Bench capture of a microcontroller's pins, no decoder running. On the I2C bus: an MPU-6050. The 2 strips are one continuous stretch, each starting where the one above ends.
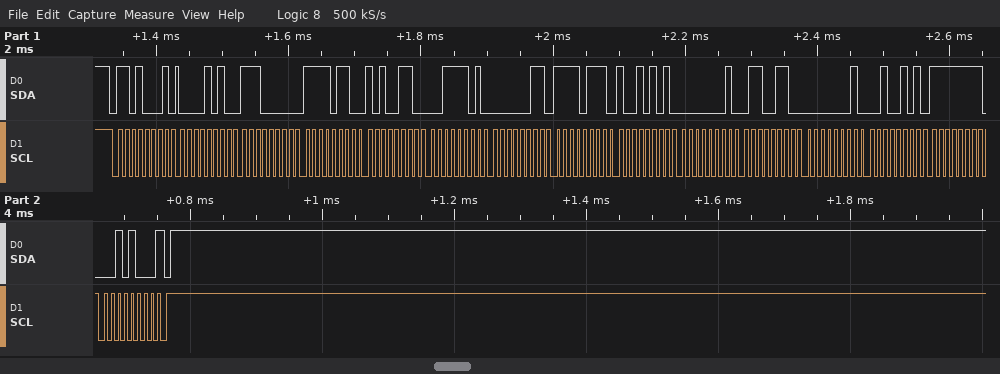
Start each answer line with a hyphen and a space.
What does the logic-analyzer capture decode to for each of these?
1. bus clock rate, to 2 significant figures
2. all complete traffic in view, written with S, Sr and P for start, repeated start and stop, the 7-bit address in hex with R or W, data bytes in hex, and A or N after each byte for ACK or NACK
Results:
- 100 kHz
- S 68R A 0A A E0 A F6 A A6 A 3D A 03 A F7 A 95 A 01 A 66 A 01 A 25 A FF A 28 N P
